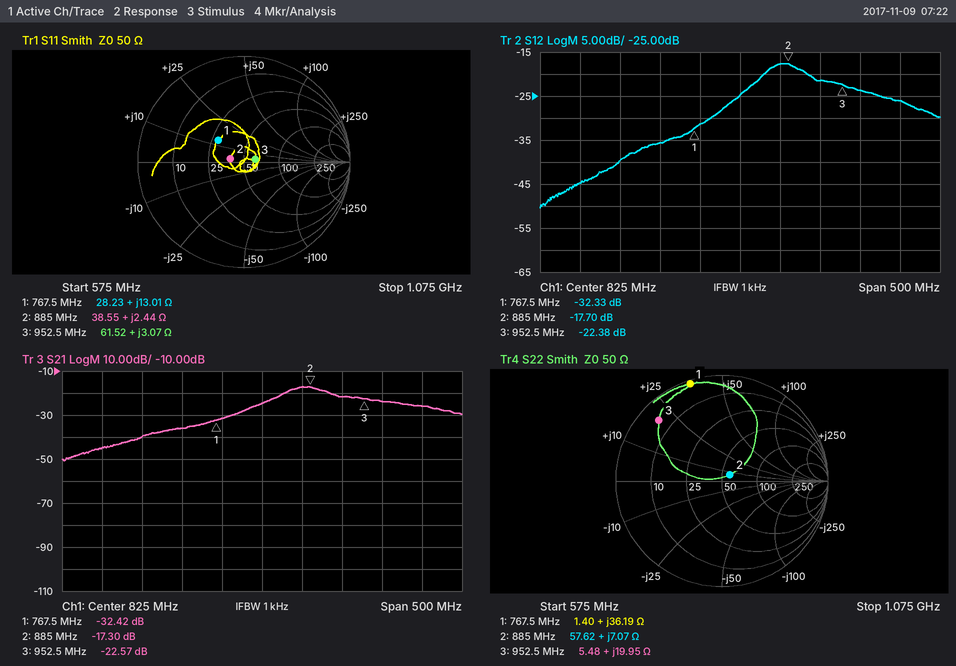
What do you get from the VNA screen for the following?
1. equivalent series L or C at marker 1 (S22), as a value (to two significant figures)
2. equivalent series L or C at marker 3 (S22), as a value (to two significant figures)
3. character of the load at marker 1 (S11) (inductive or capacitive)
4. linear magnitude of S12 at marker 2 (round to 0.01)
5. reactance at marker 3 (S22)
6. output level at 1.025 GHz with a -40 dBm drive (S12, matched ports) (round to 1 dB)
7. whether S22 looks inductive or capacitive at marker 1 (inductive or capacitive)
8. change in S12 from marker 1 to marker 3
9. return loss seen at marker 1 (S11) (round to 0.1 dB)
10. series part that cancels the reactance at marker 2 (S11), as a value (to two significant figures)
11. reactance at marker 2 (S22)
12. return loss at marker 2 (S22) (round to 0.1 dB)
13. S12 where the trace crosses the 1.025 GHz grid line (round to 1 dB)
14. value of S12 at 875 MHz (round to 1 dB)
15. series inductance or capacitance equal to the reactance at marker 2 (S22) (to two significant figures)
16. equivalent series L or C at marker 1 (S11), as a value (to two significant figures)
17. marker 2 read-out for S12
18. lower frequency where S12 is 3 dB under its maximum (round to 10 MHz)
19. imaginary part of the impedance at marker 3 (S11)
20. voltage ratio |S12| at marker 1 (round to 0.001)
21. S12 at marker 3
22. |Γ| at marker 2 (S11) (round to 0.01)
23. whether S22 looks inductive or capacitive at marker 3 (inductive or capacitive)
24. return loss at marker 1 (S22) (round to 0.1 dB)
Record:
7.5 nH
3.3 nH
inductive
0.13
+19.95 Ω
-66 dBm
inductive
9.95 dB
9.9 dB
74 pF
+7.07 Ω
20.3 dB
-26 dB
-18 dB
1.3 nH
2.7 nH
-17.70 dB
850 MHz
+3.07 Ω
0.024
-22.38 dB
0.13
inductive
0.3 dB
